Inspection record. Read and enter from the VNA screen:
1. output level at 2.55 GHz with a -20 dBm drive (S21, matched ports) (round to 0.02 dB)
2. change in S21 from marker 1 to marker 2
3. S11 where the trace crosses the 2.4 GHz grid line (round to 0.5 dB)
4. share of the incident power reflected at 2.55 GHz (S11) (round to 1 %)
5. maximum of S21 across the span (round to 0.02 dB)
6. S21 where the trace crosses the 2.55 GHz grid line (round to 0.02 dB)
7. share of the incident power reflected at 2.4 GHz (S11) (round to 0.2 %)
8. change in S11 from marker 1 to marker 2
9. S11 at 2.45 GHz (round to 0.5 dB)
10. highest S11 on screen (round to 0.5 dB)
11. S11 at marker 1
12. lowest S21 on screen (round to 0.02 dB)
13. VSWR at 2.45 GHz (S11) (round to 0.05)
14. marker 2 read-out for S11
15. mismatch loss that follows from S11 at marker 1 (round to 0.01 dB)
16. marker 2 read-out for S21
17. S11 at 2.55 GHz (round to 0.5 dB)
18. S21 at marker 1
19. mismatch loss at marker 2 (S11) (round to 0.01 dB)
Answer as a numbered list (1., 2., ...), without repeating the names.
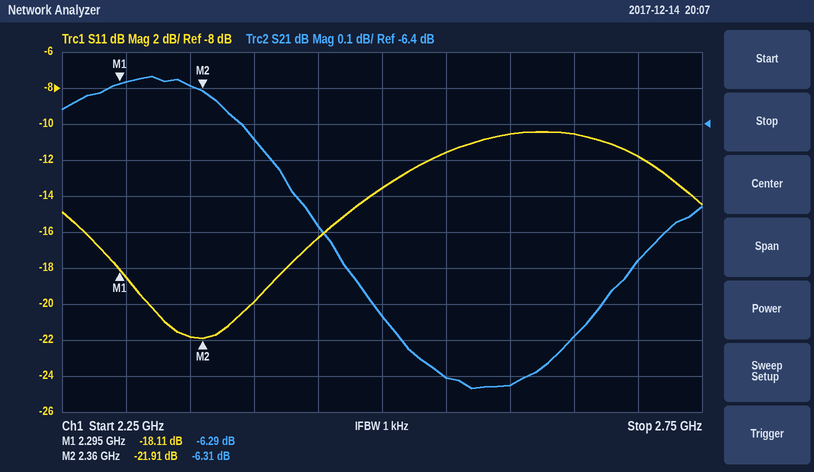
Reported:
1. -27.10 dBm
2. -0.02 dB
3. -20.0 dB
4. 7 %
5. -6.26 dB
6. -7.10 dB
7. 1.0 %
8. -3.80 dB
9. -16.5 dB
10. -10.5 dB
11. -18.11 dB
12. -7.14 dB
13. 1.35
14. -21.91 dB
15. 0.07 dB
16. -6.31 dB
17. -11.5 dB
18. -6.29 dB
19. 0.03 dB
